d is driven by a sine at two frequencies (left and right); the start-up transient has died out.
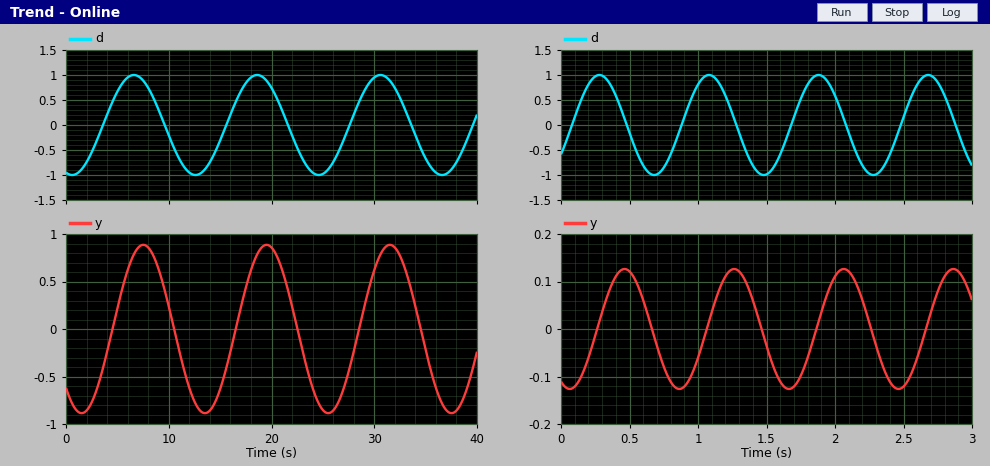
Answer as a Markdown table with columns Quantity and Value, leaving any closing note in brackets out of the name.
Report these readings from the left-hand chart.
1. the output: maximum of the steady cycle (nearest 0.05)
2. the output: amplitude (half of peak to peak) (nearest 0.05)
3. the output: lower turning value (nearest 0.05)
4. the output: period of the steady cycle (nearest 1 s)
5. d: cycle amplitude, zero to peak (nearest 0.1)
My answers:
| Quantity | Value |
|---|---|
| the output: maximum of the steady cycle | 0.90 |
| the output: amplitude (half of peak to peak) | 0.90 |
| the output: lower turning value | -0.90 |
| the output: period of the steady cycle | 12 s |
| d: cycle amplitude, zero to peak | 1.0 |
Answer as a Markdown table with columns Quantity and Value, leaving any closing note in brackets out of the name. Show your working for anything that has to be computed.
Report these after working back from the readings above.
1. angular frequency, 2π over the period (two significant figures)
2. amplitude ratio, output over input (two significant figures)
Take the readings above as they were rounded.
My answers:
| Quantity | Value |
|---|---|
| angular frequency, 2π over the period | 2π / 12 = 0.52 rad/s |
| amplitude ratio, output over input | 0.9 / 1 = 0.90 |
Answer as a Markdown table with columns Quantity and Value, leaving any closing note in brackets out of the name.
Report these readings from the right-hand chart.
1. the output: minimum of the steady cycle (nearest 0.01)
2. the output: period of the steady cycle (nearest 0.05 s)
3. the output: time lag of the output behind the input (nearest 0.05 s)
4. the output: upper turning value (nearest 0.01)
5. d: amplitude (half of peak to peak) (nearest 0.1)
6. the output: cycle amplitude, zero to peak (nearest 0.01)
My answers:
| Quantity | Value |
|---|---|
| the output: minimum of the steady cycle | -0.13 |
| the output: period of the steady cycle | 0.80 s |
| the output: time lag of the output behind the input | 0.20 s |
| the output: upper turning value | 0.13 |
| d: amplitude (half of peak to peak) | 1.0 |
| the output: cycle amplitude, zero to peak | 0.13 |
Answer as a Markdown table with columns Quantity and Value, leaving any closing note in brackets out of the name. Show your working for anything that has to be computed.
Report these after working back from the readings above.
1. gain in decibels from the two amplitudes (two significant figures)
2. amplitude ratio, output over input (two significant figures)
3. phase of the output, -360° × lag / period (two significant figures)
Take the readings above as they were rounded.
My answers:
| Quantity | Value |
|---|---|
| gain in decibels from the two amplitudes | 20 log10(0.13 / 1) = -18 dB |
| amplitude ratio, output over input | 0.13 / 1 = 0.13 |
| phase of the output, -360° × lag / period | -360 × 0.2 / 0.8 = -90° |
